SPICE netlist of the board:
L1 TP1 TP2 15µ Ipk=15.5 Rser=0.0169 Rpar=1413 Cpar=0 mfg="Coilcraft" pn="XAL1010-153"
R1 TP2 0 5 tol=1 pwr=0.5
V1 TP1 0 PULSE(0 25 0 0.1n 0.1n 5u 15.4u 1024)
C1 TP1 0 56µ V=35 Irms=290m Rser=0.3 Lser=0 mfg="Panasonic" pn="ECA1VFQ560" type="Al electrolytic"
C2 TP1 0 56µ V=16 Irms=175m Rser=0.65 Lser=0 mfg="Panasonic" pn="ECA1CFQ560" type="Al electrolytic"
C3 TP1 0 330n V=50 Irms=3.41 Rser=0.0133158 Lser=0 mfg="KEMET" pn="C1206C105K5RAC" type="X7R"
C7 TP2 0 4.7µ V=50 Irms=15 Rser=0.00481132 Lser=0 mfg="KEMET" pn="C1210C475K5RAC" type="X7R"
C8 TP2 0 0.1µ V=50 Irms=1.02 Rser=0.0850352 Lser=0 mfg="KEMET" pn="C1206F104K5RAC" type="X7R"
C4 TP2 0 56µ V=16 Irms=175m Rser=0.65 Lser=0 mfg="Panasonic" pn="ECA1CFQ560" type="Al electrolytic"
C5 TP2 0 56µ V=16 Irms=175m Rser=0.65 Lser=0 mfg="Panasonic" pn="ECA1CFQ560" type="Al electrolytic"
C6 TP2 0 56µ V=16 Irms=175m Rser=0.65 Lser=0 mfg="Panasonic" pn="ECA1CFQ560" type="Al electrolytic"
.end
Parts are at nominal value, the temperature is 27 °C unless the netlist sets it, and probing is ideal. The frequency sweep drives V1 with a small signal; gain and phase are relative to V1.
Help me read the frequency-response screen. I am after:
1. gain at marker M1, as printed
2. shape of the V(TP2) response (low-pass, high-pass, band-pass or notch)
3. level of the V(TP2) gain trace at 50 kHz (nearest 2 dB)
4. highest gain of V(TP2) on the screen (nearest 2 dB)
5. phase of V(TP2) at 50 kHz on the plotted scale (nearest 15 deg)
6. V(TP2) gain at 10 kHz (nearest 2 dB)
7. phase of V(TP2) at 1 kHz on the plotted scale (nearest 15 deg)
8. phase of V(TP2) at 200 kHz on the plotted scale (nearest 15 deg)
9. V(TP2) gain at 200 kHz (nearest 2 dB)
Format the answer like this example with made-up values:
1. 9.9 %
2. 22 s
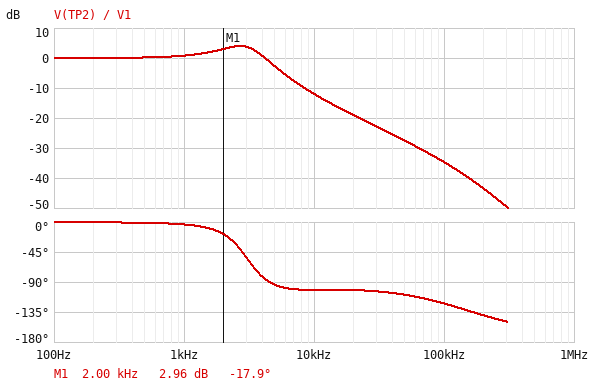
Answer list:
1. 2.96 dB
2. low-pass
3. -28 dB
4. 4 dB
5. -105 deg
6. -12 dB
7. 0 deg
8. -135 deg
9. -44 dB
